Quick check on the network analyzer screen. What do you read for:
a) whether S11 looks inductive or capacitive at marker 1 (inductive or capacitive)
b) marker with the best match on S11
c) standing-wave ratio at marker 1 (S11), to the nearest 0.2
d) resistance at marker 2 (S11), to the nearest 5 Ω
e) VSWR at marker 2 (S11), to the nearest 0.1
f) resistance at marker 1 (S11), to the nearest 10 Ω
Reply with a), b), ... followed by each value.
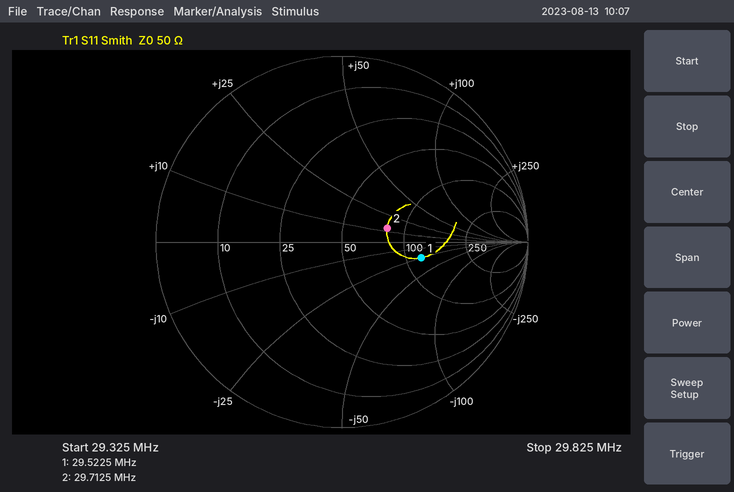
a) capacitive
b) marker 2
c) 2.6
d) 80 Ω
e) 1.7
f) 120 Ω
